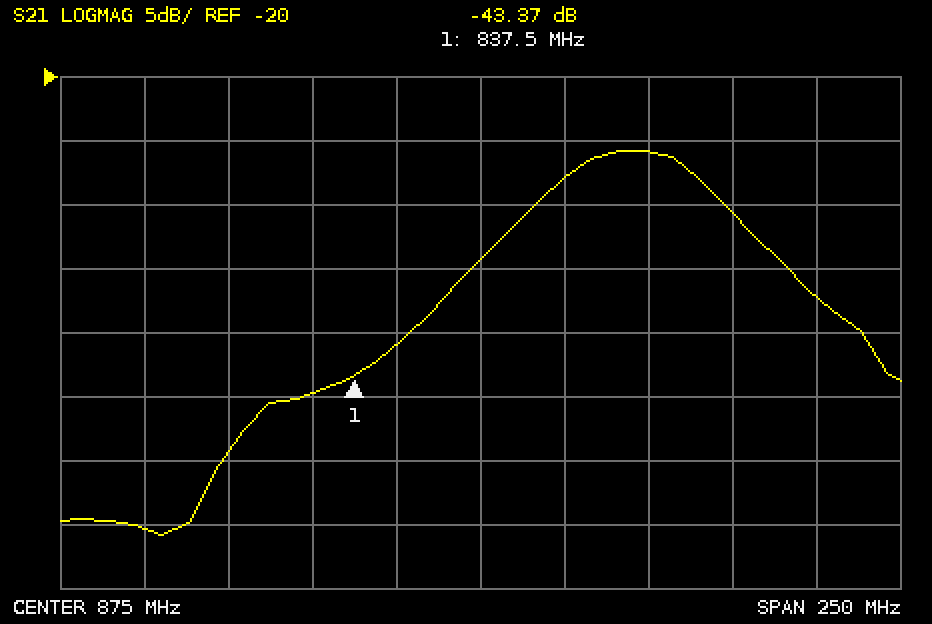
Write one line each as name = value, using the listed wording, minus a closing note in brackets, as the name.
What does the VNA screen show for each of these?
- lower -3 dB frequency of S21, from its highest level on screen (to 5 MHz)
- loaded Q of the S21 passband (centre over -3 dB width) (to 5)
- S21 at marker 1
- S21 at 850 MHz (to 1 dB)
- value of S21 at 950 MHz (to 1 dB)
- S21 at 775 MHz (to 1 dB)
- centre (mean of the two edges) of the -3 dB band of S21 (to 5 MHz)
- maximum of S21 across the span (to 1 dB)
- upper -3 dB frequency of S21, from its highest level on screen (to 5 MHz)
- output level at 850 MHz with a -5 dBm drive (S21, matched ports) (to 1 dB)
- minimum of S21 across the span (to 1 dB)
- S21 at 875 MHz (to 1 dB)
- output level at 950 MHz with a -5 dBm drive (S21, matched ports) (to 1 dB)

lower -3 dB frequency of S21, from its highest level on screen = 895 MHz
loaded Q of the S21 passband (centre over -3 dB width) = 20
S21 at marker 1 = -43.37 dB
S21 at 850 MHz = -41 dB
value of S21 at 950 MHz = -31 dB
S21 at 775 MHz = -55 dB
centre (mean of the two edges) of the -3 dB band of S21 = 920 MHz
maximum of S21 across the span = -26 dB
upper -3 dB frequency of S21, from its highest level on screen = 945 MHz
output level at 850 MHz with a -5 dBm drive (S21, matched ports) = -46 dBm
minimum of S21 across the span = -56 dB
S21 at 875 MHz = -34 dB
output level at 950 MHz with a -5 dBm drive (S21, matched ports) = -36 dBm
